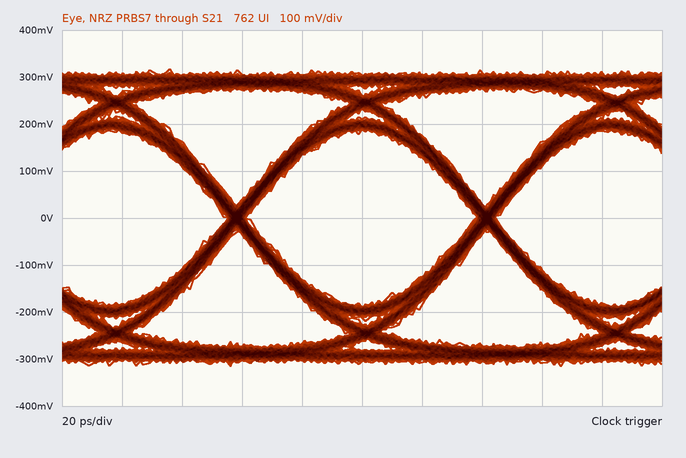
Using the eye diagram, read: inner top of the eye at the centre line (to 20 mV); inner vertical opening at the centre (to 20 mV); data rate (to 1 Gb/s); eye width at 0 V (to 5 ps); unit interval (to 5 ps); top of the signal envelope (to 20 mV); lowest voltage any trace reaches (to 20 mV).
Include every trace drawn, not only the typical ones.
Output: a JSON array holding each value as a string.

["180 mV", "380 mV", "12 Gb/s", "75 ps", "85 ps", "320 mV", "-320 mV"]
